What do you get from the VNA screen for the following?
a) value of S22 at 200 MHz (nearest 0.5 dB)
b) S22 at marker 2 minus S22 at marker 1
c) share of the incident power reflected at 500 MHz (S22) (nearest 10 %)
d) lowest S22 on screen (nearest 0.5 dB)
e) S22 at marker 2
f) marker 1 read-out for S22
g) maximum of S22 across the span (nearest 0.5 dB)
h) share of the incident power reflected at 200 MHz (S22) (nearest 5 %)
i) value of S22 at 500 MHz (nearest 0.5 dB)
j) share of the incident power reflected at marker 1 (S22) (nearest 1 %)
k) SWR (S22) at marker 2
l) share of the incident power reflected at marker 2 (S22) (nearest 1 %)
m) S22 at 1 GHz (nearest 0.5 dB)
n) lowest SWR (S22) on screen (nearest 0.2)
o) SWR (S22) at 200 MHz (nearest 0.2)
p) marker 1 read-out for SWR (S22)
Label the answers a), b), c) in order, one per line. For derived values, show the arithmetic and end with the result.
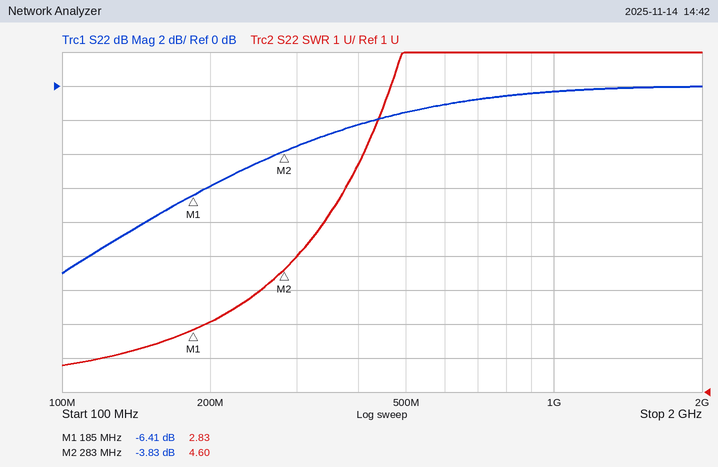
a) -6.0 dB
b) -3.83 − (-6.41) = 2.58 dB
c) 10^(-1.5/10) ≈ 70.8 %, so 70 % to the nearest 10 %
d) -11.0 dB
e) -3.83 dB
f) -6.41 dB
g) 0.0 dB
h) 10^(-6/10) ≈ 25 %
i) -1.5 dB
j) 10^(-6.41/10) ≈ 23 %
k) 4.60
l) 10^(-3.83/10) ≈ 41 %
m) -0.5 dB
n) 1.8
o) 3.0
p) 2.83
